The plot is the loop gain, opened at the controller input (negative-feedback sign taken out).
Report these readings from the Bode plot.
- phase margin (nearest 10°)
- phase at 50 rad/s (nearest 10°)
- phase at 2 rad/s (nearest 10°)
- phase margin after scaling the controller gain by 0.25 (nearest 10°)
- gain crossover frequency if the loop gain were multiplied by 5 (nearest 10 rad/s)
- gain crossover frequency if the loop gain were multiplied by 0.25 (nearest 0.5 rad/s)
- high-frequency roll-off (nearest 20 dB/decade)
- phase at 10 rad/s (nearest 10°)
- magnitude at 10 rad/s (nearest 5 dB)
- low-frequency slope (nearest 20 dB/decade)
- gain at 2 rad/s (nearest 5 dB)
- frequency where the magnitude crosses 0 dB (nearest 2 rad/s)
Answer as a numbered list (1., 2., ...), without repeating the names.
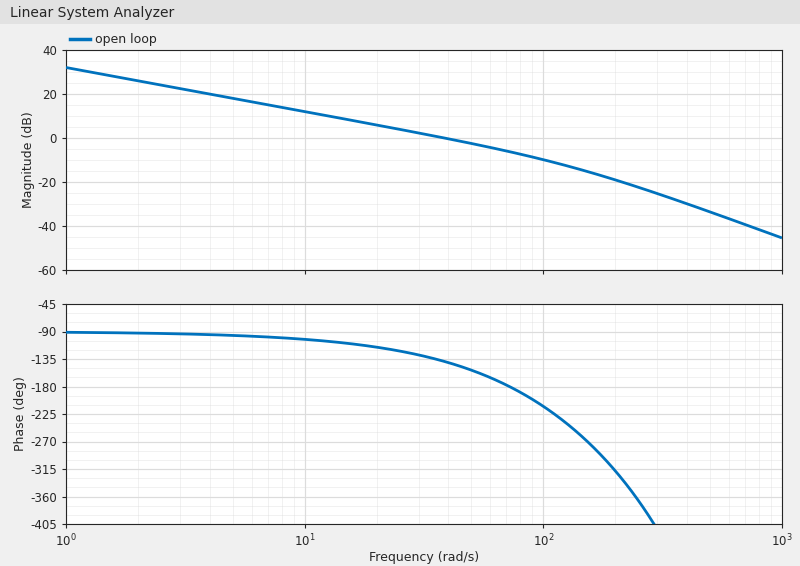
1. 40°
2. -150°
3. -90°
4. 80°
5. 140 rad/s
6. 10.0 rad/s
7. -40 dB/decade
8. -100°
9. 10 dB
10. -20 dB/decade
11. 25 dB
12. 38 rad/s
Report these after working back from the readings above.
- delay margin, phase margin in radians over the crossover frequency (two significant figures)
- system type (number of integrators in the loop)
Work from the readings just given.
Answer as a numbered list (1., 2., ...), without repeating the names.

1. 0.018 s
2. 1
